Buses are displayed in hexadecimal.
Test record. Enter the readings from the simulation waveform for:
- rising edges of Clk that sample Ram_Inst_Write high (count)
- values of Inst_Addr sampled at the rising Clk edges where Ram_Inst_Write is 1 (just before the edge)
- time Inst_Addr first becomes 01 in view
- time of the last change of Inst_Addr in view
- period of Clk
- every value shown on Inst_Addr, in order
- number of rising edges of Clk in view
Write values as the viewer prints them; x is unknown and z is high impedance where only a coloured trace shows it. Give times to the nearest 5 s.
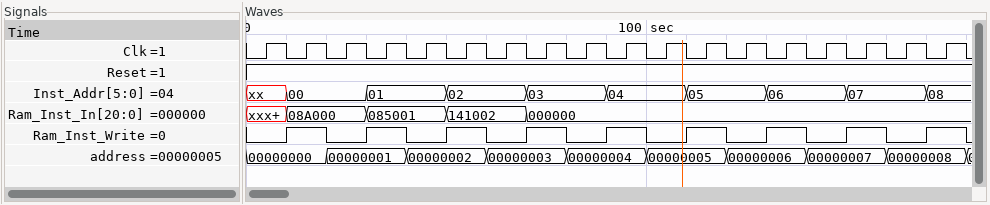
9
00, 01, 02, 03, 04, 05, 06, 07, 08
30 s
170 s
10 s
xx, 00, 01, 02, 03, 04, 05, 06, 07, 08
18
